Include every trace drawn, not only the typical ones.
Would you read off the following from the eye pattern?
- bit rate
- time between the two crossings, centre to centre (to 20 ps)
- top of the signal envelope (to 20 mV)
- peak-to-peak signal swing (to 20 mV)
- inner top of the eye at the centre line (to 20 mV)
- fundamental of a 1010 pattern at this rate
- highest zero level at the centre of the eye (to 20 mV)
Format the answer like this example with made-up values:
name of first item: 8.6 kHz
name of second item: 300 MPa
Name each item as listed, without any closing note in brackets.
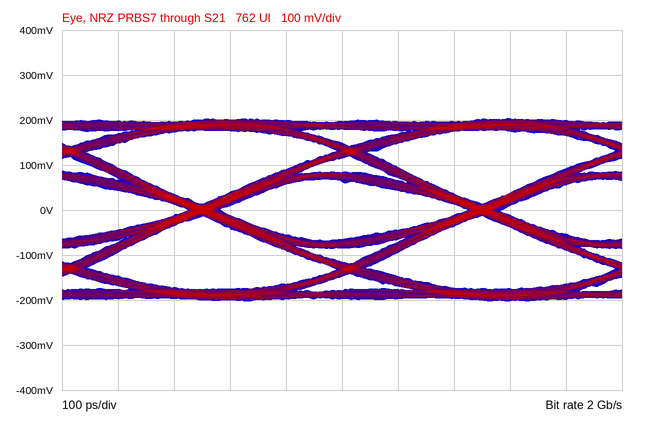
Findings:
bit rate: 2 Gb/s
time between the two crossings, centre to centre: 500 ps
top of the signal envelope: 200 mV
peak-to-peak signal swing: 400 mV
inner top of the eye at the centre line: 60 mV
fundamental of a 1010 pattern at this rate: 1 GHz
highest zero level at the centre of the eye: -60 mV
